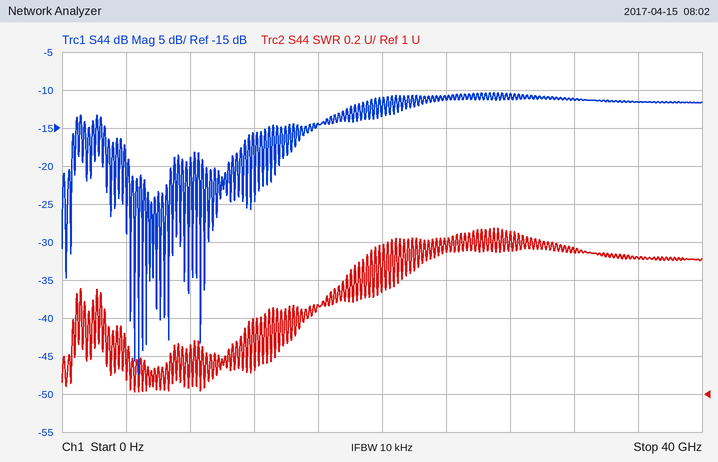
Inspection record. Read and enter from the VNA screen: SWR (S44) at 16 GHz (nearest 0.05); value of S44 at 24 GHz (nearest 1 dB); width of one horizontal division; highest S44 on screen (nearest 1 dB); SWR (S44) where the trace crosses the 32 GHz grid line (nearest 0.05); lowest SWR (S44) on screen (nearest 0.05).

1.45
-11 dB
4 GHz
-10 dB
1.75
1.00
